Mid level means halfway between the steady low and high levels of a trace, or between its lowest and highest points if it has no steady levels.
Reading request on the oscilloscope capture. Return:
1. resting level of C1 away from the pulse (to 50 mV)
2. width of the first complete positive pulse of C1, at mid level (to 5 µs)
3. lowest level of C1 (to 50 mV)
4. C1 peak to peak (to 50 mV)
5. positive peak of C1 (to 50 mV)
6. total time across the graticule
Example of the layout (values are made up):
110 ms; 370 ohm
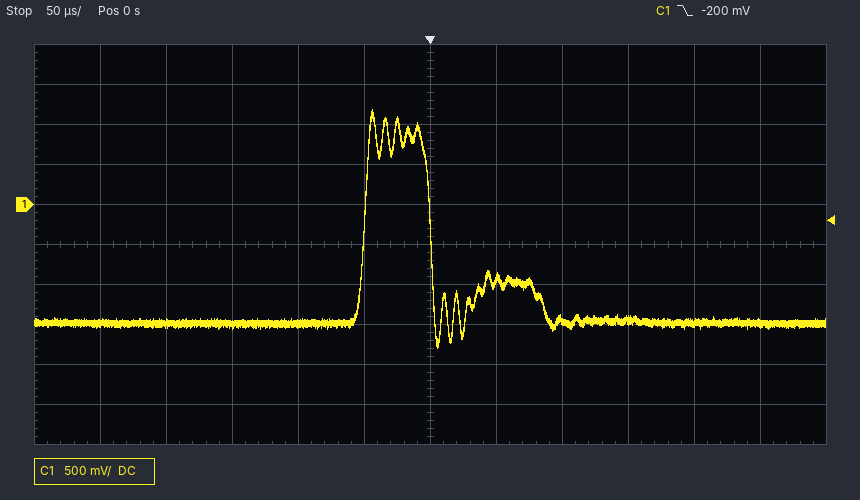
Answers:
-1.50 V; 50 µs; -1.80 V; 3.00 V; 1.20 V; 600 µs
